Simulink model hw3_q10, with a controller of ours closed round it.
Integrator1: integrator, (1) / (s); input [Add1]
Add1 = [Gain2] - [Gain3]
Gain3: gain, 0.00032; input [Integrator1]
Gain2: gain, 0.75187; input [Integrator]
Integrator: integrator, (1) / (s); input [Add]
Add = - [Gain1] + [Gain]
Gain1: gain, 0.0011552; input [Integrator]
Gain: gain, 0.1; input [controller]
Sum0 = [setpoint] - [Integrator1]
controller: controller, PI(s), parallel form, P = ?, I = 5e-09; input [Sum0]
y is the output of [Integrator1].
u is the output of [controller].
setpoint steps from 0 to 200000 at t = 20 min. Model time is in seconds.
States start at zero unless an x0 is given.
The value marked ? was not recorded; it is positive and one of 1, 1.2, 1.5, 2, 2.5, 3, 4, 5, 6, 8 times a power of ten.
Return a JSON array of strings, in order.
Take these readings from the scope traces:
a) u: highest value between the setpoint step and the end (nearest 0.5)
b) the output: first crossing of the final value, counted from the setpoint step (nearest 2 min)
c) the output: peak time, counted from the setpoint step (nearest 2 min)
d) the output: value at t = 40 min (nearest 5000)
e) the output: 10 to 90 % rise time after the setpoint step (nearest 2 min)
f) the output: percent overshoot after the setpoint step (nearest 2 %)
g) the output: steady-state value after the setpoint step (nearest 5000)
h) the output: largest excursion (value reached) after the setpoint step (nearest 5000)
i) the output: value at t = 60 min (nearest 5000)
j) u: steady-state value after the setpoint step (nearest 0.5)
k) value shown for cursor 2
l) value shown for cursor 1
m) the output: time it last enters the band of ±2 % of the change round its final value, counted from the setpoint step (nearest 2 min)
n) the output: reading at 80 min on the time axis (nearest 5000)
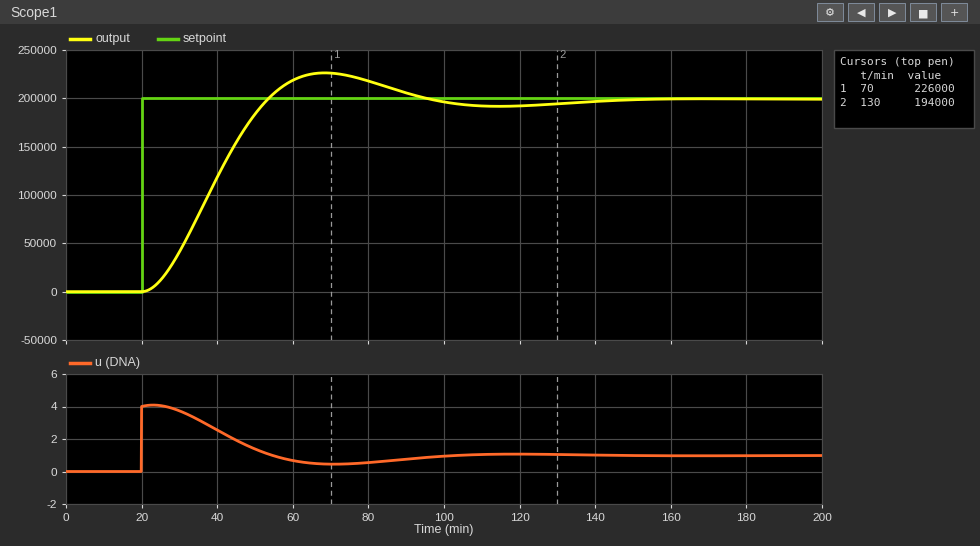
["4.0", "34 min", "48 min", "120000", "22 min", "14 %", "200000", "225000", "220000", "1.0", "194000", "226000", "116 min", "220000"]
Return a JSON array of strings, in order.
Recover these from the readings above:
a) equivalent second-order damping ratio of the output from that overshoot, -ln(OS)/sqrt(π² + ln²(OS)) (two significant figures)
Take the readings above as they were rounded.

["0.53"]
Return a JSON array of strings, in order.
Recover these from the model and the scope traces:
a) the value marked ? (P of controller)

["2e-05"]
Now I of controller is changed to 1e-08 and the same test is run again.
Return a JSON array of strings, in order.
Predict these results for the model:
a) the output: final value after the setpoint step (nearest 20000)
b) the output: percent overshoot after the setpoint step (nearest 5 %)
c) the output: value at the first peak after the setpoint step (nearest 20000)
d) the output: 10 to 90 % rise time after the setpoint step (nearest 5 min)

["200000", "30 %", "260000", "20 min"]
